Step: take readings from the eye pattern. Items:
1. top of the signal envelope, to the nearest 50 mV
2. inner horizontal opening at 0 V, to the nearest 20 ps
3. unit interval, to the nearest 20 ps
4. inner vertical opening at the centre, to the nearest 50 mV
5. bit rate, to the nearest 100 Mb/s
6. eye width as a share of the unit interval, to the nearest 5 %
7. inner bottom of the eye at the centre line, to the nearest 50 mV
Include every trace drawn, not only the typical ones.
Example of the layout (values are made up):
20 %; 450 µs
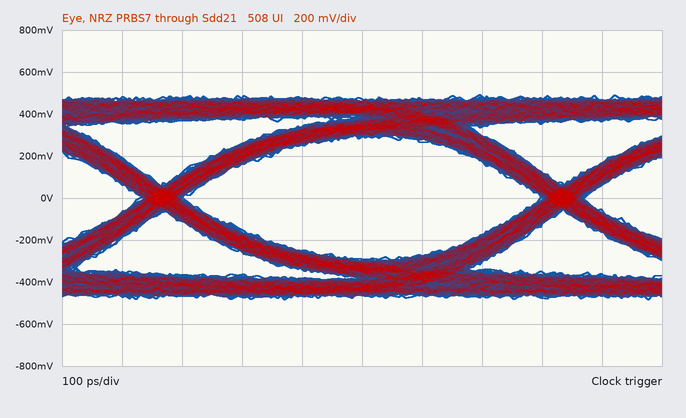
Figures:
500 mV; 600 ps; 660 ps; 600 mV; 1.5 Gb/s; 90 %; -300 mV
